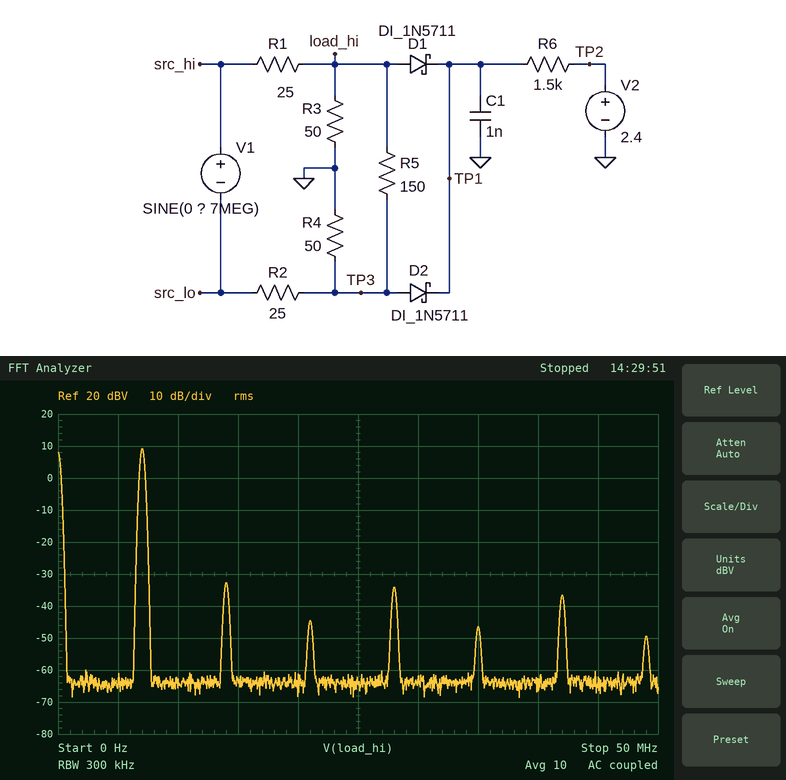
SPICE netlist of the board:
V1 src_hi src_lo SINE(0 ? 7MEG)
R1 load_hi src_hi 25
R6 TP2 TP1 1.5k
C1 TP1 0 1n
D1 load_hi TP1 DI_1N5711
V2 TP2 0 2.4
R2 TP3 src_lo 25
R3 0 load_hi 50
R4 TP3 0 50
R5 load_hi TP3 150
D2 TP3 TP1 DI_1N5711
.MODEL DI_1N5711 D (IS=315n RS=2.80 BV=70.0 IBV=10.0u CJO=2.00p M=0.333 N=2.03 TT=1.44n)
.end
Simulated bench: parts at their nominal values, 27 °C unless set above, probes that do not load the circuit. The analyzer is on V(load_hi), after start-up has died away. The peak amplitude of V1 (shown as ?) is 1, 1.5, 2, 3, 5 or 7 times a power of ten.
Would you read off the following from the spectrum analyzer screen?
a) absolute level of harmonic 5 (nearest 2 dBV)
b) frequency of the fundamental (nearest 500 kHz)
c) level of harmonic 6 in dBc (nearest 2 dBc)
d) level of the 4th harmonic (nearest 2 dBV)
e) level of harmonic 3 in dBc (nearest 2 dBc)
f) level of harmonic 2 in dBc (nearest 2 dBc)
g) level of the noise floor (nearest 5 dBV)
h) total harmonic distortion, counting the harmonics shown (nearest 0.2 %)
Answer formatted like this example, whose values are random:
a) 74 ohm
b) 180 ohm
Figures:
a) -46 dBV
b) 7.0 MHz
c) -46 dBc
d) -34 dBV
e) -54 dBc
f) -42 dBc
g) -65 dBV
h) 1.2 %
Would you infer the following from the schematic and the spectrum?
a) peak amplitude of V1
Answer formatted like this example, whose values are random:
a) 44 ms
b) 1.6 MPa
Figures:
a) 15 V
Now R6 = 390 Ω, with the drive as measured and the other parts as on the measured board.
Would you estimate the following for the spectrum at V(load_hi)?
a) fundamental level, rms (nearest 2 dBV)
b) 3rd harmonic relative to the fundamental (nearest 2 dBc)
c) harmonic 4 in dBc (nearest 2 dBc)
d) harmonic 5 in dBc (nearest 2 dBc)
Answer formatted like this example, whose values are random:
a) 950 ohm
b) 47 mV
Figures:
a) 10 dBV
b) -46 dBc
c) -36 dBc
d) -48 dBc
